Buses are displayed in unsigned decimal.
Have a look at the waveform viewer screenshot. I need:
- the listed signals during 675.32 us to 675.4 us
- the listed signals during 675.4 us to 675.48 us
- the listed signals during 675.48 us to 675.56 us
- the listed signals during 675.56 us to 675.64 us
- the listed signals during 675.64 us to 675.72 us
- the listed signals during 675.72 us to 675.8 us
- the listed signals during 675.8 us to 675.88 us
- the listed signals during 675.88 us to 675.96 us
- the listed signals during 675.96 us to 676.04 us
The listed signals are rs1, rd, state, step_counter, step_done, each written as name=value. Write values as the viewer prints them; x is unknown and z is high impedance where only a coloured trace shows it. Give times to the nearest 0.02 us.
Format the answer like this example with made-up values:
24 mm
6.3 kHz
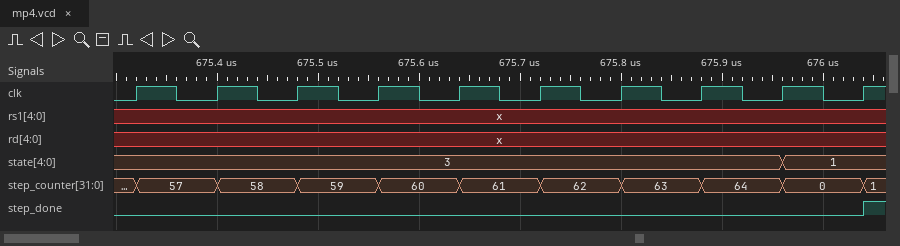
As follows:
rs1=x, rd=x, state=3, step_counter=57, step_done=0
rs1=x, rd=x, state=3, step_counter=58, step_done=0
rs1=x, rd=x, state=3, step_counter=59, step_done=0
rs1=x, rd=x, state=3, step_counter=60, step_done=0
rs1=x, rd=x, state=3, step_counter=61, step_done=0
rs1=x, rd=x, state=3, step_counter=62, step_done=0
rs1=x, rd=x, state=3, step_counter=63, step_done=0
rs1=x, rd=x, state=3, step_counter=64, step_done=0
rs1=x, rd=x, state=1, step_counter=0, step_done=0
